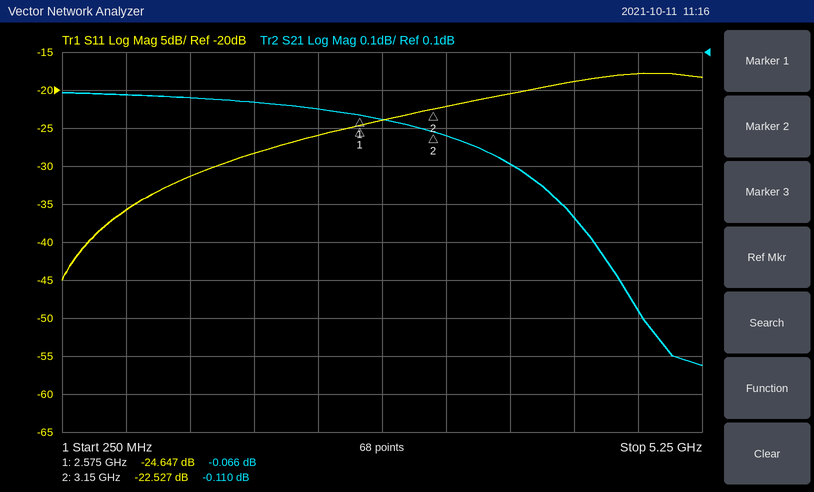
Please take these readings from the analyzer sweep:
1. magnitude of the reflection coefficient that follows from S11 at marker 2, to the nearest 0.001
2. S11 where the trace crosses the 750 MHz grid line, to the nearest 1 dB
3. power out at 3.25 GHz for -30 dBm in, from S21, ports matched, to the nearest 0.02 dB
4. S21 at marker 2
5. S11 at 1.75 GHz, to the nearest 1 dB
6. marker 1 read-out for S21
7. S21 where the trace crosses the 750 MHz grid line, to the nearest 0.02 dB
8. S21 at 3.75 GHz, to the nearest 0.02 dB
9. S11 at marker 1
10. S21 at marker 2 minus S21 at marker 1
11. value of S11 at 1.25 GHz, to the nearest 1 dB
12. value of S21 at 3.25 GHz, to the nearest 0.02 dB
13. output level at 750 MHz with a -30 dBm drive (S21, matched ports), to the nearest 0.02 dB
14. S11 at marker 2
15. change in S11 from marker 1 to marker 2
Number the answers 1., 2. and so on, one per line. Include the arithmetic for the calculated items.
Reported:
1. 10^(-22.527/20) ≈ 0.075
2. -36 dB
3. -30 dBm + (-0.12 dB) = -30.12 dBm
4. -0.110 dB
5. -28 dB
6. -0.066 dB
7. -0.02 dB
8. -0.20 dB
9. -24.647 dB
10. -0.11 − (-0.066) = -0.044 dB
11. -31 dB
12. -0.12 dB
13. -30 dBm + (-0.02 dB) = -30.02 dBm
14. -22.527 dB
15. -22.527 − (-24.647) = 2.120 dB
